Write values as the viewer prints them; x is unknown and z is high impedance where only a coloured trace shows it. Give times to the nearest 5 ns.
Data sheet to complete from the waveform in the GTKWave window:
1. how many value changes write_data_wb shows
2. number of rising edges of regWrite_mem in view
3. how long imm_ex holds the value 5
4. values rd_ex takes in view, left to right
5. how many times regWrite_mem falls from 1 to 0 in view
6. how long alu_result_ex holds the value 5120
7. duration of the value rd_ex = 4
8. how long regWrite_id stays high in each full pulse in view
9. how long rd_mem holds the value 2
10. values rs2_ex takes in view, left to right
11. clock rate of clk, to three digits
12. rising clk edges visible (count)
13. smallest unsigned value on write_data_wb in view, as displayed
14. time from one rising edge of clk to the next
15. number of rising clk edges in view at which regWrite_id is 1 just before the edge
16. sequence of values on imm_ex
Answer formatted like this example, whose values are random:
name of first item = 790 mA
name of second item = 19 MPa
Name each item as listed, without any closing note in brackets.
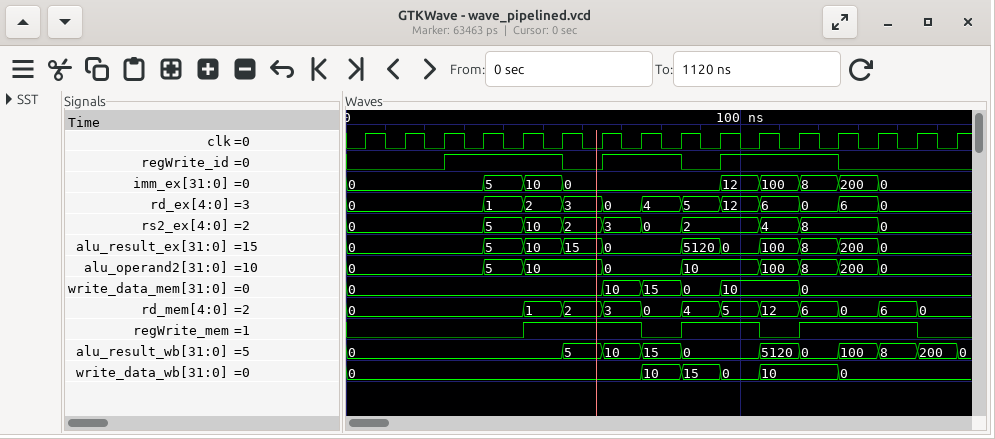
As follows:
how many value changes write_data_wb shows = 5
number of rising edges of regWrite_mem in view = 3
how long imm_ex holds the value 5 = 10 ns
values rd_ex takes in view, left to right = 0, 1, 2, 3, 0, 4, 5, 12, 6, 0, 6, 0
how many times regWrite_mem falls from 1 to 0 in view = 3
how long alu_result_ex holds the value 5120 = 10 ns
duration of the value rd_ex = 4 = 10 ns
how long regWrite_id stays high in each full pulse in view = 30 ns, 20 ns, 30 ns
how long rd_mem holds the value 2 = 10 ns
values rs2_ex takes in view, left to right = 0, 5, 10, 2, 3, 0, 2, 4, 8, 0
clock rate of clk, to three digits = 100 MHz
rising clk edges visible = 16
smallest unsigned value on write_data_wb in view, as displayed = 0
time from one rising edge of clk to the next = 10 ns
number of rising clk edges in view at which regWrite_id is 1 just before the edge = 8
sequence of values on imm_ex = 0, 5, 10, 0, 12, 100, 8, 200, 0
